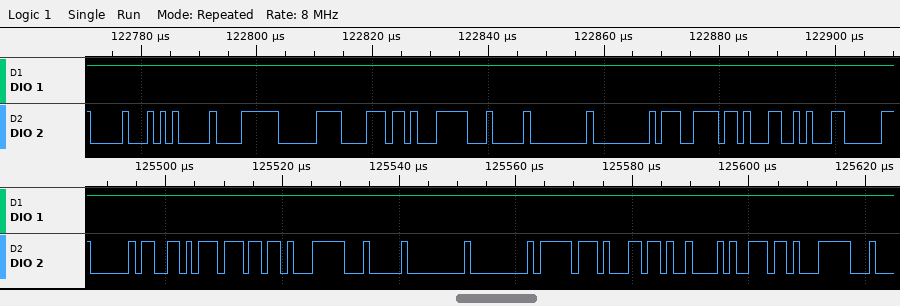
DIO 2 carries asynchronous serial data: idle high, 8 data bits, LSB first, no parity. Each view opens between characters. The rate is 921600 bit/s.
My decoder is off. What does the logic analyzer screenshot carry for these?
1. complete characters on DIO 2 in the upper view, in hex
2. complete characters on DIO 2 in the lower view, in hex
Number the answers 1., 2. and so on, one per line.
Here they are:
1. 10, 05, F8, E0, B8, F1, 04, 00, 00, E7, 8B, 8A
2. A0, D6, B7, F1, 04, 00, 00, DF, B1, 09, B9, F1
